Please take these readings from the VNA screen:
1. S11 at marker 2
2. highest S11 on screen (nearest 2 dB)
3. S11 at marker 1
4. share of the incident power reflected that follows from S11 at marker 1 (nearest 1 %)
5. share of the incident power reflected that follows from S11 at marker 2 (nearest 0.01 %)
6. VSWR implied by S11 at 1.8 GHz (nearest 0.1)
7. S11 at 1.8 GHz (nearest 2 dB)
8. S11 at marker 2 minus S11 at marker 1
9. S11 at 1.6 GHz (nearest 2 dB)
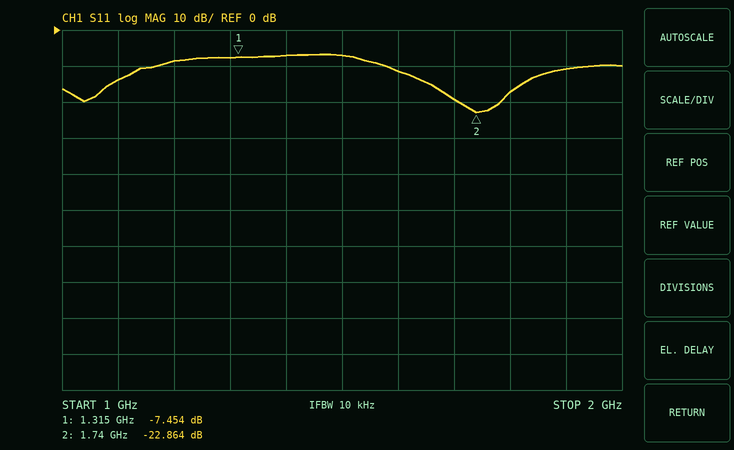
-22.864 dB
-6 dB
-7.454 dB
18 %
0.52 %
1.3
-18 dB
-15.410 dB
-12 dB
